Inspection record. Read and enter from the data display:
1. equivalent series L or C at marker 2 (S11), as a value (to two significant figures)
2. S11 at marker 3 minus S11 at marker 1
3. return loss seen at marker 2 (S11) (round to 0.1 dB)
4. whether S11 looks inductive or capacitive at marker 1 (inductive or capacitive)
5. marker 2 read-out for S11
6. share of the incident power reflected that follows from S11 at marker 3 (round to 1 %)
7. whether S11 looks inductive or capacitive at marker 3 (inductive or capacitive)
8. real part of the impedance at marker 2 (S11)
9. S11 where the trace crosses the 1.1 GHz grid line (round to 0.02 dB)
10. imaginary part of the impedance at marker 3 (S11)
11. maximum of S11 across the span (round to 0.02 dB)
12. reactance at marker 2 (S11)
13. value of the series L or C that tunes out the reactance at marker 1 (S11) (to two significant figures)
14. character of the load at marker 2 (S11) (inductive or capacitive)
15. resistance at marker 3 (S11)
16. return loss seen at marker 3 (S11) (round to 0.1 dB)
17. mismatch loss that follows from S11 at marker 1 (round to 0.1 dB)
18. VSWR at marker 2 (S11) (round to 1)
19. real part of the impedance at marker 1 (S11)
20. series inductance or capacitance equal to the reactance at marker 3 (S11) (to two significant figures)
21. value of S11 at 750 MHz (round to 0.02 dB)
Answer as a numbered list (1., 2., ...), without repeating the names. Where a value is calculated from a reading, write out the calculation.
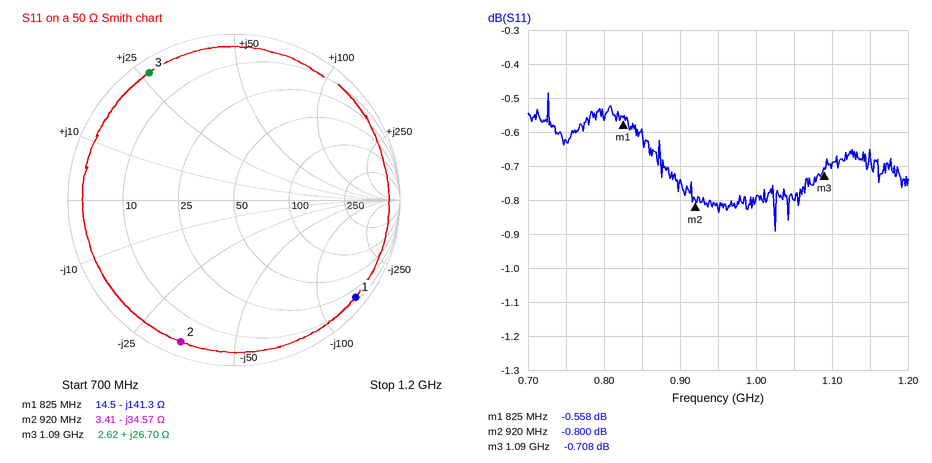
1. C = 1/(2π × 920 MHz × 34.57 Ω) ≈ 5.0 pF
2. -0.708 − (-0.558) = -0.150 dB
3. 0.8 dB
4. capacitive
5. -0.800 dB
6. 10^(-0.708/10) ≈ 85 %
7. inductive
8. 3.41 Ω
9. -0.70 dB
10. +26.70 Ω
11. -0.48 dB
12. -34.57 Ω
13. L = 141.3 Ω/(2π × 825 MHz) ≈ 27 nH
14. capacitive
15. 2.62 Ω
16. 0.7 dB
17. −10 log10(1 − 10^(-0.558/10)) ≈ 9.2 dB
18. (1 + 0.9120)/(1 − 0.9120) ≈ 22
19. 14.5 Ω
20. L = 26.7 Ω/(2π × 1.09 GHz) ≈ 3.9 nH
21. -0.62 dB
